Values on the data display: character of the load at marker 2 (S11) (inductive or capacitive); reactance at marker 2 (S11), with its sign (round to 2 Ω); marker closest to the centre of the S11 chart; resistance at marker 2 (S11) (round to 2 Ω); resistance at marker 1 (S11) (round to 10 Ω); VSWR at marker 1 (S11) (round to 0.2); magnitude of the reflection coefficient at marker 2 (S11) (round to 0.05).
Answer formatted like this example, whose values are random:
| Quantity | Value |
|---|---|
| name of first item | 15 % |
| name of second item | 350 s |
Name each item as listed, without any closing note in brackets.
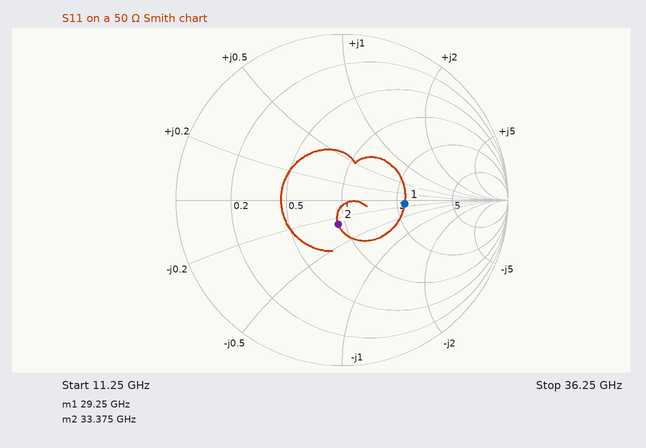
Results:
| Quantity | Value |
|---|---|
| character of the load at marker 2 (S11) | capacitive |
| reactance at marker 2 (S11), with its sign | -14 Ω |
| marker closest to the centre of the S11 chart | marker 2 |
| resistance at marker 2 (S11) | 46 Ω |
| resistance at marker 1 (S11) | 110 Ω |
| VSWR at marker 1 (S11) | 2.2 |
| magnitude of the reflection coefficient at marker 2 (S11) | 0.15 |
